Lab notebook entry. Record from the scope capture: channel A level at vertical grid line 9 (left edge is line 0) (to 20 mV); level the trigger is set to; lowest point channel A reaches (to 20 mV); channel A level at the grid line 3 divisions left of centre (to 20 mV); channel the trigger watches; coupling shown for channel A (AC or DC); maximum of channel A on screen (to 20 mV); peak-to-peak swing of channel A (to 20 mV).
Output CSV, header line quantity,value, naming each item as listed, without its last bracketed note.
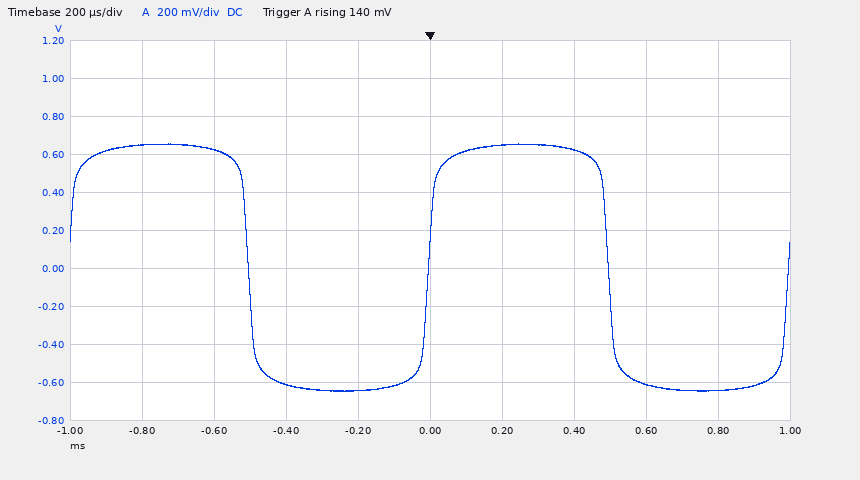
quantity,value
channel A level at vertical grid line 9 (left edge is line 0),-640 mV
level the trigger is set to,140 mV
lowest point channel A reaches,-640 mV
channel A level at the grid line 3 divisions left of centre,620 mV
channel the trigger watches,channel A
coupling shown for channel A,DC
maximum of channel A on screen,660 mV
peak-to-peak swing of channel A,1.30 V
